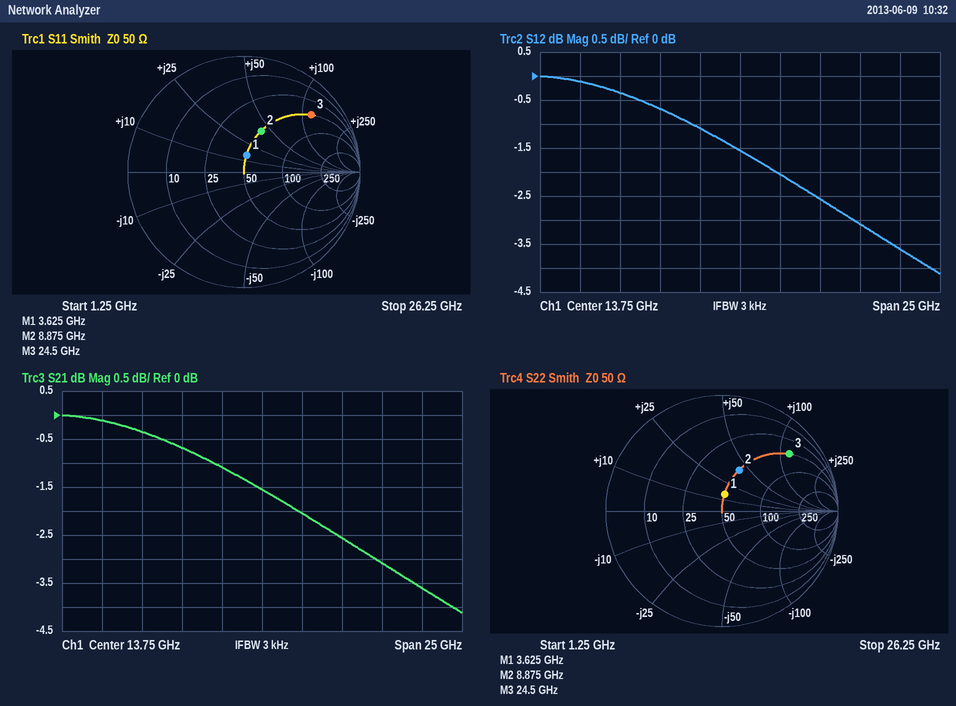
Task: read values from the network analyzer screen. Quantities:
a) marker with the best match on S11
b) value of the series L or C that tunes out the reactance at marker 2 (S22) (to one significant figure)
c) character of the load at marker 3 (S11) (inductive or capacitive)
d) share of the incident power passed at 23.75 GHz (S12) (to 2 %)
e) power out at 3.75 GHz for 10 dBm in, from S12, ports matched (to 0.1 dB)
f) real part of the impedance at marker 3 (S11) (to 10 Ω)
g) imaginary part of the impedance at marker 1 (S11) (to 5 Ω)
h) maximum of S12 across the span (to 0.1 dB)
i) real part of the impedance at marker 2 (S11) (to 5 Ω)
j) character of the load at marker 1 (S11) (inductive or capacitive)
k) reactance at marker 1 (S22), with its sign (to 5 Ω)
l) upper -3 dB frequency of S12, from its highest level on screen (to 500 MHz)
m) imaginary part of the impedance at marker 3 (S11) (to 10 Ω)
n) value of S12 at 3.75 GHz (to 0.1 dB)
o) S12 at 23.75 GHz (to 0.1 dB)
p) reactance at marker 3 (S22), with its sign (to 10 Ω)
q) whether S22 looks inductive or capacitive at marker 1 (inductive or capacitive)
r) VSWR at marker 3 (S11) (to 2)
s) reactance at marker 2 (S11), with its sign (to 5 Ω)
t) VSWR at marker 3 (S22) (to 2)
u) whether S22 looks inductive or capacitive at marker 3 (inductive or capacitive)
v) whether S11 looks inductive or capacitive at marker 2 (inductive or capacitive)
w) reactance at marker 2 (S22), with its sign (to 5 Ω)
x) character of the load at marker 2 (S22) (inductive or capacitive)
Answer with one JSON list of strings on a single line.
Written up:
["marker 1", "400 fF", "inductive", "44 %", "9.9 dBm", "50 Ω", "+15 Ω", "0.0 dB", "50 Ω", "inductive", "+15 Ω", "21.0 GHz", "+120 Ω", "-0.1 dB", "-3.6 dB", "+120 Ω", "inductive", "8", "+40 Ω", "8", "inductive", "inductive", "+40 Ω", "inductive"]
